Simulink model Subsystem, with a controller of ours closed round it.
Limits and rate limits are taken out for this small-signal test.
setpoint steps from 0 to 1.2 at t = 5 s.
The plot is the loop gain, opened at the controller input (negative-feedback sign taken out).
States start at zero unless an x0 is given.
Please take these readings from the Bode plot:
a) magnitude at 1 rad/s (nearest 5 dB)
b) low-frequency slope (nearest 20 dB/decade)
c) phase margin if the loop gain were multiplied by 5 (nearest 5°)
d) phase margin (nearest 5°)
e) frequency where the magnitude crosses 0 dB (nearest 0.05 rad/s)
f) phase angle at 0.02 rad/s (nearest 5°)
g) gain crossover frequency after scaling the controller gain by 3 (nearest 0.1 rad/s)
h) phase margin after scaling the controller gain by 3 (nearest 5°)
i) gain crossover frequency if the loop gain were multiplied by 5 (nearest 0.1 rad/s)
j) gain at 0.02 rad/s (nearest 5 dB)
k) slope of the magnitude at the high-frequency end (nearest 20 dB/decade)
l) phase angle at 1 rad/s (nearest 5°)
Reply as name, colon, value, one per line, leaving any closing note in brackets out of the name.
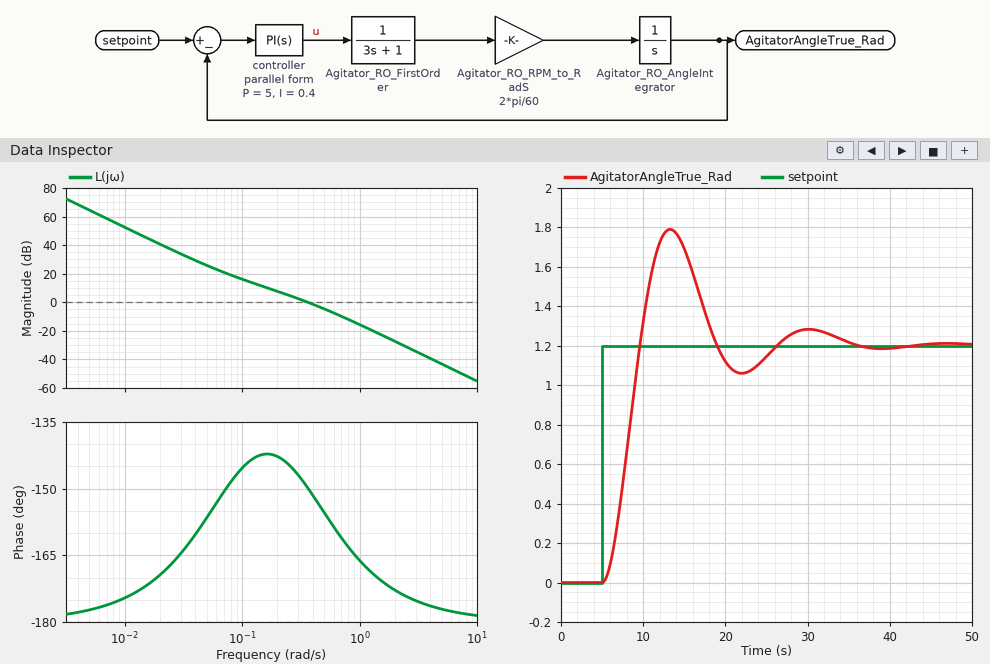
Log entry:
magnitude at 1 rad/s: -15 dB
low-frequency slope: -40 dB/decade
phase margin if the loop gain were multiplied by 5: 15°
phase margin: 30°
frequency where the magnitude crosses 0 dB: 0.35 rad/s
phase angle at 0.02 rad/s: -170°
gain crossover frequency after scaling the controller gain by 3: 0.7 rad/s
phase margin after scaling the controller gain by 3: 20°
gain crossover frequency if the loop gain were multiplied by 5: 0.9 rad/s
gain at 0.02 rad/s: 40 dB
slope of the magnitude at the high-frequency end: -40 dB/decade
phase angle at 1 rad/s: -165°
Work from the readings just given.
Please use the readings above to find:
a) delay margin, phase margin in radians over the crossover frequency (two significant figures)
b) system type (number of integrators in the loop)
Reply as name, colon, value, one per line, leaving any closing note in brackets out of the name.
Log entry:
delay margin, phase margin in radians over the crossover frequency: 1.5 s
system type: 2
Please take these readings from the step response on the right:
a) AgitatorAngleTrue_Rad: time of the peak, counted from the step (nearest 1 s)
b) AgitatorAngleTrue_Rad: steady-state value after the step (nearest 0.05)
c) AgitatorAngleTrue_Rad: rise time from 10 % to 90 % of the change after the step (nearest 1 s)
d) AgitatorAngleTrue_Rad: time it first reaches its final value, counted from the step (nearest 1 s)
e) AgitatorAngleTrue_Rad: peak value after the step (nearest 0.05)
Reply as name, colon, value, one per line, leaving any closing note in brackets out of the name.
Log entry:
AgitatorAngleTrue_Rad: time of the peak, counted from the step: 8 s
AgitatorAngleTrue_Rad: steady-state value after the step: 1.20
AgitatorAngleTrue_Rad: rise time from 10 % to 90 % of the change after the step: 3 s
AgitatorAngleTrue_Rad: time it first reaches its final value, counted from the step: 5 s
AgitatorAngleTrue_Rad: peak value after the step: 1.80
